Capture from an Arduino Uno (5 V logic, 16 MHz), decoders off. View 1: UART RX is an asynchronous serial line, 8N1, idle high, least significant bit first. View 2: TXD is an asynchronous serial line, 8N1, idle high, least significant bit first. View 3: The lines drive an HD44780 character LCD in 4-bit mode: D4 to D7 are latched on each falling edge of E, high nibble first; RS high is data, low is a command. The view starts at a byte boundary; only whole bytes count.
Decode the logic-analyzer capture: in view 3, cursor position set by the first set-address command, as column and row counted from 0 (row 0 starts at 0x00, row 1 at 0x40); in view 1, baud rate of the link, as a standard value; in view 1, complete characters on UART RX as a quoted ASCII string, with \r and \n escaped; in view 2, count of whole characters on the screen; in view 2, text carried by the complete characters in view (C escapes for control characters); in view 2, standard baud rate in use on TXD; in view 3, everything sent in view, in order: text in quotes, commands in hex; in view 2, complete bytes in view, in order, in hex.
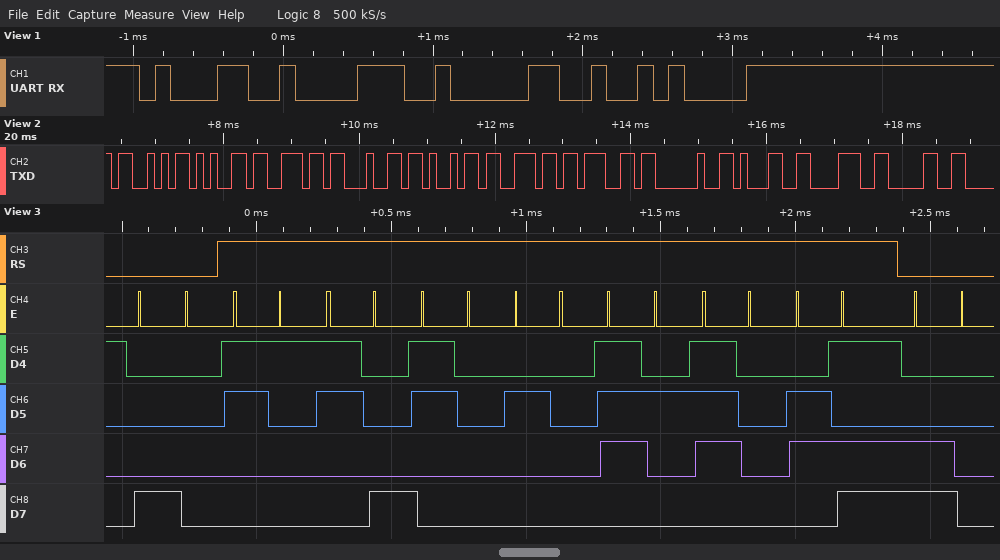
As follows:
column 0, row 0
9600 baud
"180\n"
11
"Sending 180"
9600 baud
0x80 "180 rpm" 0xC0
53 65 6E 64 69 6E 67 20 31 38 30
